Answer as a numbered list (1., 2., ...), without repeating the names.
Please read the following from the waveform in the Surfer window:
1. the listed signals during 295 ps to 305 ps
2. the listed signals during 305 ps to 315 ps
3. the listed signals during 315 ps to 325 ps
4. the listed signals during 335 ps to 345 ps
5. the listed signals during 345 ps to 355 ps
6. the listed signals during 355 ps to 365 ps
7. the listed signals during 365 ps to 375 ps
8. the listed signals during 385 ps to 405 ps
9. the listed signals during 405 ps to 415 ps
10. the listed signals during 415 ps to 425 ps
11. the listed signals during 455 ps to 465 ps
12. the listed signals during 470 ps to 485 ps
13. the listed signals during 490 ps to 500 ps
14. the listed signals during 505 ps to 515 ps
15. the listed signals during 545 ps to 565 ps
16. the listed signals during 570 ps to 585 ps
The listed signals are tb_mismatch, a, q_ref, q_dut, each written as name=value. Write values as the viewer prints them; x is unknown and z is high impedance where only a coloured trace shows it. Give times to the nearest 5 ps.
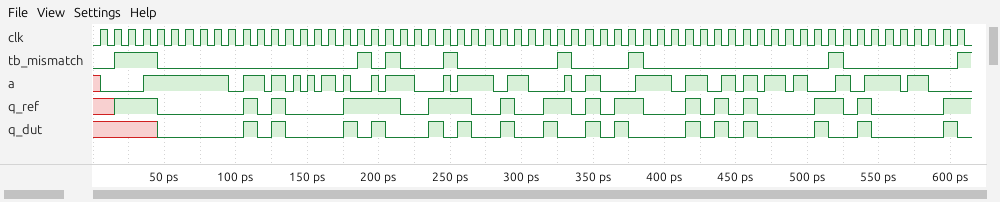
1. tb_mismatch=0, a=1, q_ref=0, q_dut=0
2. tb_mismatch=0, a=0, q_ref=0, q_dut=0
3. tb_mismatch=0, a=0, q_ref=1, q_dut=1
4. tb_mismatch=0, a=0, q_ref=0, q_dut=0
5. tb_mismatch=0, a=1, q_ref=1, q_dut=1
6. tb_mismatch=0, a=0, q_ref=0, q_dut=0
7. tb_mismatch=0, a=0, q_ref=1, q_dut=1
8. tb_mismatch=0, a=1, q_ref=0, q_dut=0
9. tb_mismatch=0, a=0, q_ref=0, q_dut=0
10. tb_mismatch=0, a=1, q_ref=1, q_dut=1
11. tb_mismatch=0, a=1, q_ref=1, q_dut=1
12. tb_mismatch=0, a=1, q_ref=0, q_dut=0
13. tb_mismatch=0, a=1, q_ref=0, q_dut=0
14. tb_mismatch=0, a=0, q_ref=1, q_dut=1
15. tb_mismatch=0, a=1, q_ref=0, q_dut=0
16. tb_mismatch=0, a=1, q_ref=0, q_dut=0
